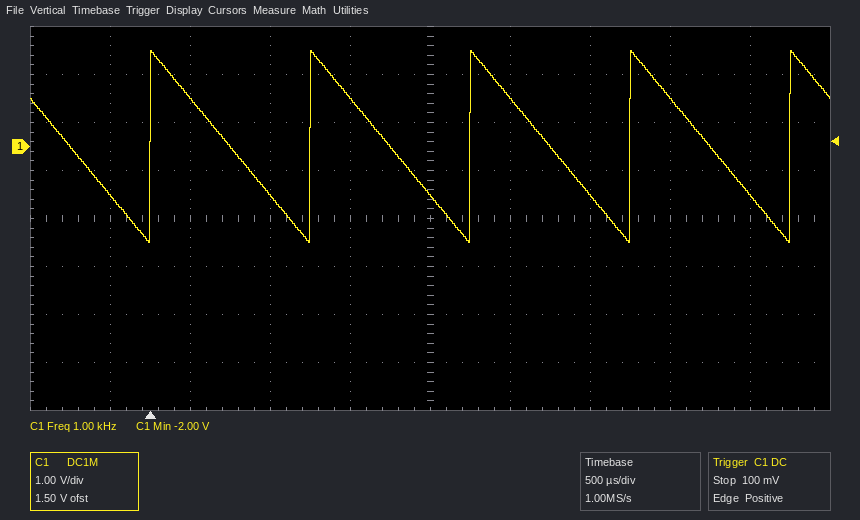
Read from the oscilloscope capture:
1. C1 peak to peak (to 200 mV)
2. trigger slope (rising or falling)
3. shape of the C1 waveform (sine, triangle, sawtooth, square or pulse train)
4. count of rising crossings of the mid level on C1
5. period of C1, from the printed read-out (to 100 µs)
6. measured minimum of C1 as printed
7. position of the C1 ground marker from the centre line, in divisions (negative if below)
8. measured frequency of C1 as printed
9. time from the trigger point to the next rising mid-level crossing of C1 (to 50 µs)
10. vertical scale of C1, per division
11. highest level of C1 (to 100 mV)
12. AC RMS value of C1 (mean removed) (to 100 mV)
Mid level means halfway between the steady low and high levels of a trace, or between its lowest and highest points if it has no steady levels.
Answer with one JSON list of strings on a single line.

["4.0 V", "rising", "sawtooth", "5", "1.0 ms", "-2.00 V", "+1.5 div", "1.00 kHz", "1.00 ms", "1 V", "2.0 V", "1.2 V"]
